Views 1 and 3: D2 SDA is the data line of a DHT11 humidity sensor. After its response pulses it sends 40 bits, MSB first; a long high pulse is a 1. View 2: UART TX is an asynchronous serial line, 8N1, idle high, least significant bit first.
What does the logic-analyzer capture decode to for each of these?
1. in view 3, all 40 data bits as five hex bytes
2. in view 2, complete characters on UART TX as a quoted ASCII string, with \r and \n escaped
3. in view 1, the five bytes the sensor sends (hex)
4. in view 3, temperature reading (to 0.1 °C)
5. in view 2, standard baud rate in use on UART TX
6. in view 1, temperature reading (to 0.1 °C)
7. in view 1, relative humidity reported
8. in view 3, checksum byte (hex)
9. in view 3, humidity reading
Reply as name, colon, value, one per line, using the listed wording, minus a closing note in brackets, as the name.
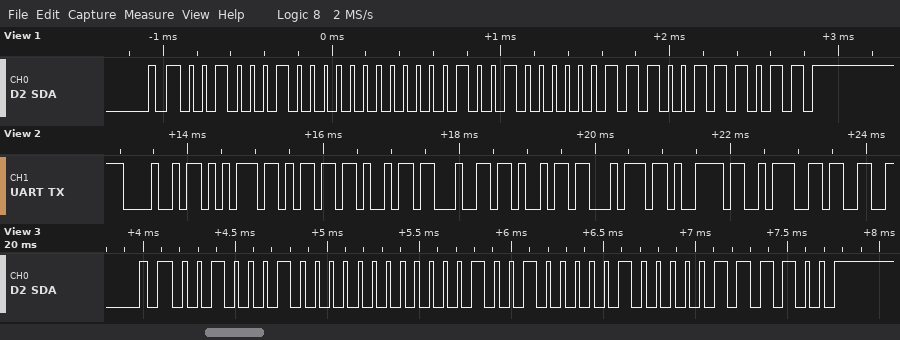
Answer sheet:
in view 3, all 40 data bits as five hex bytes: 22 00 12 08 3C
in view 2, complete characters on UART TX as a quoted ASCII string, with \r and \n escaped: "Humidity:3"
in view 1, the five bytes the sensor sends: 22 00 12 07 3B
in view 3, temperature reading: 18.8 °C
in view 2, standard baud rate in use on UART TX: 9600 baud
in view 1, temperature reading: 18.7 °C
in view 1, relative humidity reported: 34 %
in view 3, checksum byte: 0x3C
in view 3, humidity reading: 34 %
